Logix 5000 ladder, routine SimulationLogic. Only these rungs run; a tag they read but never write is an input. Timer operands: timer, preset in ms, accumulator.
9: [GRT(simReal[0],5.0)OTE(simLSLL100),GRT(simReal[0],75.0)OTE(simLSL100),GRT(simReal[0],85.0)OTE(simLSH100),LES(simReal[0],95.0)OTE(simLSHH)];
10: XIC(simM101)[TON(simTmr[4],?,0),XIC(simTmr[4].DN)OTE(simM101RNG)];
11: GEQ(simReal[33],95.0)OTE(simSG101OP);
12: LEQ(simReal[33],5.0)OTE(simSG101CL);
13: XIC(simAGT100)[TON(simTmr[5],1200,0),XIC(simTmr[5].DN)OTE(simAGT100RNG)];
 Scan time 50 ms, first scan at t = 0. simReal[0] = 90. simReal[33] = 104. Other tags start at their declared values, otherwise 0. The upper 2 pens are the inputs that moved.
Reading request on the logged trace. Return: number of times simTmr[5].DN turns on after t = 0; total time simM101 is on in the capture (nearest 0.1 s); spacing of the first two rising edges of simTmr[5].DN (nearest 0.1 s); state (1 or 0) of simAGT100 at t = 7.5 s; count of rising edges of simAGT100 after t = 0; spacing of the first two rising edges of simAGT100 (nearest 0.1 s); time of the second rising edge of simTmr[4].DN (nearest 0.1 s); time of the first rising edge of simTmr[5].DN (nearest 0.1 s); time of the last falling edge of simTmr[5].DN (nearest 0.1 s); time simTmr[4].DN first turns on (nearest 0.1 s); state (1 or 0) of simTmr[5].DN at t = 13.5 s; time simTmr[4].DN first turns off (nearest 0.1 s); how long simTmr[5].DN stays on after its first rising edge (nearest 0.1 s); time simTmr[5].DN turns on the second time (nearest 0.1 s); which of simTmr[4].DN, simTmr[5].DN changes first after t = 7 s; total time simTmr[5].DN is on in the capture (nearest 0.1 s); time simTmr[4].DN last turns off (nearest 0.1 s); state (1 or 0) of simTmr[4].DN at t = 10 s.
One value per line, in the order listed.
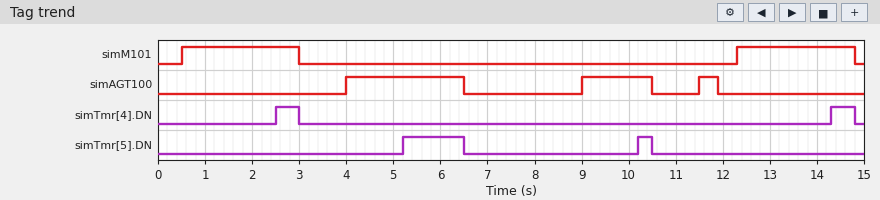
2
5.0 s
5.0 s
0
3
5.0 s
14.3 s
5.2 s
10.5 s
2.5 s
0
3.0 s
1.3 s
10.2 s
simTmr[5].DN
1.6 s
14.8 s
0
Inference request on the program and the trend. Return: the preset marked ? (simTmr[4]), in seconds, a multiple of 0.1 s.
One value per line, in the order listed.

2.0 s
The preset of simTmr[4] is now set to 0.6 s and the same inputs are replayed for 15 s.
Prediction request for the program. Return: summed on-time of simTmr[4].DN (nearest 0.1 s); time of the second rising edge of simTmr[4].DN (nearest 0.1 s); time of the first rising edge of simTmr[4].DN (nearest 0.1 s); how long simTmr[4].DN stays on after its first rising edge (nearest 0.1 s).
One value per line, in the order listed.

3.8 s
12.9 s
1.1 s
1.9 s
